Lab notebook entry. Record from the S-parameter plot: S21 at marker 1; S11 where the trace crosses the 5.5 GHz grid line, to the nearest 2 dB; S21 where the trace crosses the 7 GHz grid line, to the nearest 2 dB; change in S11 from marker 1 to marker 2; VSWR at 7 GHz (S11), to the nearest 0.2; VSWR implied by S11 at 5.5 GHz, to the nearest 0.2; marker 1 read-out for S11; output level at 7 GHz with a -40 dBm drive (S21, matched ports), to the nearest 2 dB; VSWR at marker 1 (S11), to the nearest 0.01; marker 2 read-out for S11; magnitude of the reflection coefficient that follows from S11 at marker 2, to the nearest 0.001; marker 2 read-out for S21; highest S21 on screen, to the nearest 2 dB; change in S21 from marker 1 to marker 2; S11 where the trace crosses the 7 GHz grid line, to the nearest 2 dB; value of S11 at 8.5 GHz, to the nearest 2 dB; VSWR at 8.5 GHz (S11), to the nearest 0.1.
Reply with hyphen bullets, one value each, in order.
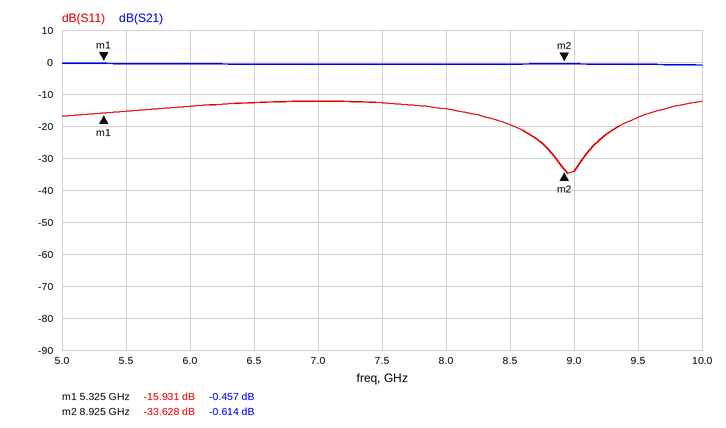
- -0.457 dB
- -16 dB
- 0 dB
- -17.697 dB
- 1.6
- 1.4
- -15.931 dB
- -40 dBm
- 1.38
- -33.628 dB
- 0.021
- -0.614 dB
- 0 dB
- -0.157 dB
- -12 dB
- -20 dB
- 1.2
